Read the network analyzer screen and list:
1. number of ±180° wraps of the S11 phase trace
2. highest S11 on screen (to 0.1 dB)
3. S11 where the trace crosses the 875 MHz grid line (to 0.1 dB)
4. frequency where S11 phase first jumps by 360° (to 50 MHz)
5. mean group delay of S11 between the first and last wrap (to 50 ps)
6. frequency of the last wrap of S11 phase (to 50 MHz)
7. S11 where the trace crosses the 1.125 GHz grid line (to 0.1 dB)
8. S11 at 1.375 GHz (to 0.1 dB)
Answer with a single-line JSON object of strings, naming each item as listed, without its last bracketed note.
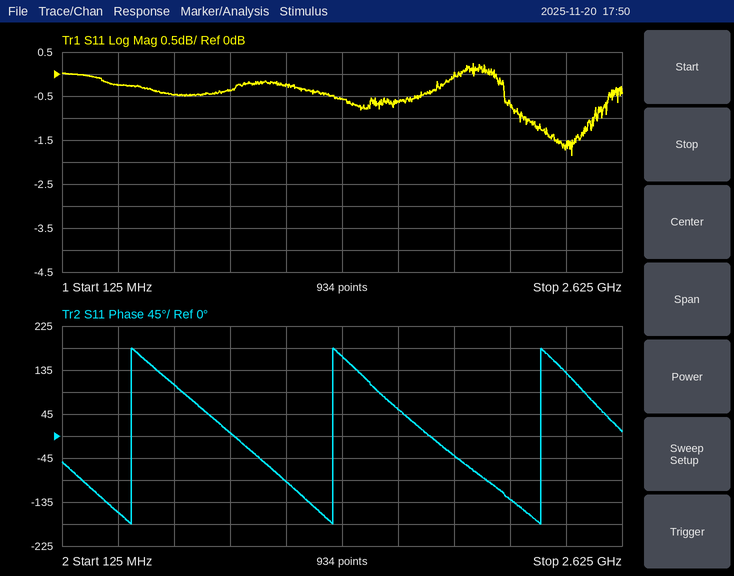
{"number of ±180° wraps of the S11 phase trace": "3", "highest S11 on screen": "0.2 dB", "S11 where the trace crosses the 875 MHz grid line": "-0.4 dB", "frequency where S11 phase first jumps by 360°": "450 MHz", "mean group delay of S11 between the first and last wrap": "1.10 ns", "frequency of the last wrap of S11 phase": "2.25 GHz", "S11 where the trace crosses the 1.125 GHz grid line": "-0.2 dB", "S11 at 1.375 GHz": "-0.6 dB"}
